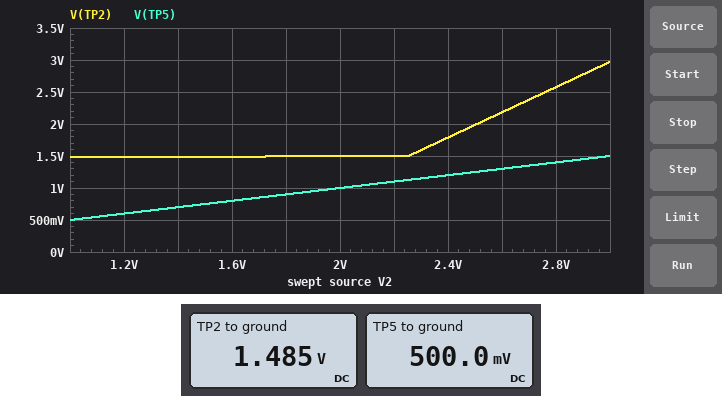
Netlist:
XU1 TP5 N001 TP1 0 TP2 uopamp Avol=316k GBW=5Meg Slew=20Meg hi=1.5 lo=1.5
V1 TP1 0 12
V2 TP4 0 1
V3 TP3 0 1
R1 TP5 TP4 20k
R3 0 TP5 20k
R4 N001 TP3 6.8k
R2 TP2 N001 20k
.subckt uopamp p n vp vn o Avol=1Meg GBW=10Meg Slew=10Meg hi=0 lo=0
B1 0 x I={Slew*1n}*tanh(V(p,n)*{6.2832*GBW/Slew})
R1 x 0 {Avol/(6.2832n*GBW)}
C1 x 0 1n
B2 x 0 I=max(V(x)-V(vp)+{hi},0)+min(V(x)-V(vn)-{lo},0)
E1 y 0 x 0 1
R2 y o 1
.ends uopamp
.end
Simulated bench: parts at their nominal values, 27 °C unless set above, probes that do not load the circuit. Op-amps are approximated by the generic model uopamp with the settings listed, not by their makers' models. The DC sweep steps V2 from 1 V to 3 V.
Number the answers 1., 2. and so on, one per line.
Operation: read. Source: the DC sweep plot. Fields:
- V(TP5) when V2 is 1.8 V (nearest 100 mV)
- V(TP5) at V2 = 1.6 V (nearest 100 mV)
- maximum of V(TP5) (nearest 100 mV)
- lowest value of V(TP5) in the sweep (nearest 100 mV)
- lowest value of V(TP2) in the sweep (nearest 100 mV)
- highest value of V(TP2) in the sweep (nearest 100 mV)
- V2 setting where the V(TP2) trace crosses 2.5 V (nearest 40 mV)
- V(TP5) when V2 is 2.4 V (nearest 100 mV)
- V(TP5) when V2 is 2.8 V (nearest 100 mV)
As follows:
1. 900 mV
2. 800 mV
3. 1.5 V
4. 500 mV
5. 1.5 V
6. 3.0 V
7. 2.76 V
8. 1.2 V
9. 1.4 V
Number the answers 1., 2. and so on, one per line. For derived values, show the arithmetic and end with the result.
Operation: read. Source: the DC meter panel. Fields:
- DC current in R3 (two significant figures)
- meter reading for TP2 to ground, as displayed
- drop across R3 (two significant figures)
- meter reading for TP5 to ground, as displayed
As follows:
1. (500 mV) / 20 kΩ = 25 µA
2. 1.485 V
3. 500 mV = 500 mV
4. 500.0 mV
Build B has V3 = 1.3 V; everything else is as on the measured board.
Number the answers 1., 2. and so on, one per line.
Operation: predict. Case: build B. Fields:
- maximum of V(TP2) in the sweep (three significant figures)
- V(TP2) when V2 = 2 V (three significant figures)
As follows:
1. 2.09 V
2. 1.49 V
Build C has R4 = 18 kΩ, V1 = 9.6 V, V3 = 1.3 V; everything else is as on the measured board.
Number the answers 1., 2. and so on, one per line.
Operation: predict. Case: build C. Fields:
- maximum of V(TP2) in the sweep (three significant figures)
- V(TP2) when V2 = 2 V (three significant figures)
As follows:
1. 1.72 V
2. 1.49 V
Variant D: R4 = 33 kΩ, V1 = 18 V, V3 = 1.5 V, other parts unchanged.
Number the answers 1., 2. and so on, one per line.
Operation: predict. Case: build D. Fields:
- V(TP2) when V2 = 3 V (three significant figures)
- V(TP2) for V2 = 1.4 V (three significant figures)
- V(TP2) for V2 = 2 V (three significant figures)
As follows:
1. 1.50 V
2. 1.48 V
3. 1.49 V
